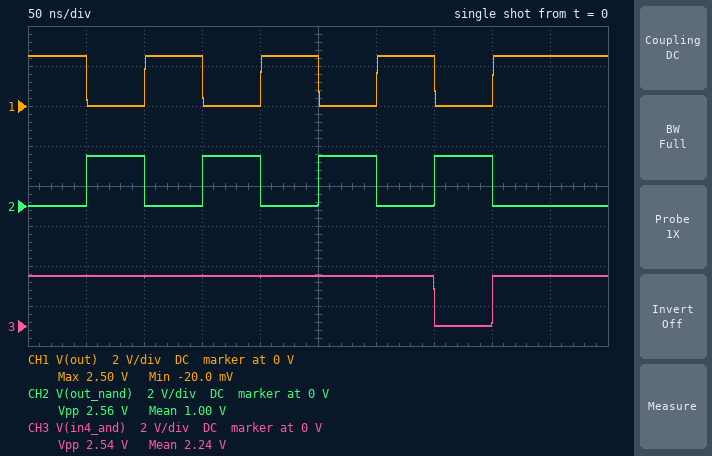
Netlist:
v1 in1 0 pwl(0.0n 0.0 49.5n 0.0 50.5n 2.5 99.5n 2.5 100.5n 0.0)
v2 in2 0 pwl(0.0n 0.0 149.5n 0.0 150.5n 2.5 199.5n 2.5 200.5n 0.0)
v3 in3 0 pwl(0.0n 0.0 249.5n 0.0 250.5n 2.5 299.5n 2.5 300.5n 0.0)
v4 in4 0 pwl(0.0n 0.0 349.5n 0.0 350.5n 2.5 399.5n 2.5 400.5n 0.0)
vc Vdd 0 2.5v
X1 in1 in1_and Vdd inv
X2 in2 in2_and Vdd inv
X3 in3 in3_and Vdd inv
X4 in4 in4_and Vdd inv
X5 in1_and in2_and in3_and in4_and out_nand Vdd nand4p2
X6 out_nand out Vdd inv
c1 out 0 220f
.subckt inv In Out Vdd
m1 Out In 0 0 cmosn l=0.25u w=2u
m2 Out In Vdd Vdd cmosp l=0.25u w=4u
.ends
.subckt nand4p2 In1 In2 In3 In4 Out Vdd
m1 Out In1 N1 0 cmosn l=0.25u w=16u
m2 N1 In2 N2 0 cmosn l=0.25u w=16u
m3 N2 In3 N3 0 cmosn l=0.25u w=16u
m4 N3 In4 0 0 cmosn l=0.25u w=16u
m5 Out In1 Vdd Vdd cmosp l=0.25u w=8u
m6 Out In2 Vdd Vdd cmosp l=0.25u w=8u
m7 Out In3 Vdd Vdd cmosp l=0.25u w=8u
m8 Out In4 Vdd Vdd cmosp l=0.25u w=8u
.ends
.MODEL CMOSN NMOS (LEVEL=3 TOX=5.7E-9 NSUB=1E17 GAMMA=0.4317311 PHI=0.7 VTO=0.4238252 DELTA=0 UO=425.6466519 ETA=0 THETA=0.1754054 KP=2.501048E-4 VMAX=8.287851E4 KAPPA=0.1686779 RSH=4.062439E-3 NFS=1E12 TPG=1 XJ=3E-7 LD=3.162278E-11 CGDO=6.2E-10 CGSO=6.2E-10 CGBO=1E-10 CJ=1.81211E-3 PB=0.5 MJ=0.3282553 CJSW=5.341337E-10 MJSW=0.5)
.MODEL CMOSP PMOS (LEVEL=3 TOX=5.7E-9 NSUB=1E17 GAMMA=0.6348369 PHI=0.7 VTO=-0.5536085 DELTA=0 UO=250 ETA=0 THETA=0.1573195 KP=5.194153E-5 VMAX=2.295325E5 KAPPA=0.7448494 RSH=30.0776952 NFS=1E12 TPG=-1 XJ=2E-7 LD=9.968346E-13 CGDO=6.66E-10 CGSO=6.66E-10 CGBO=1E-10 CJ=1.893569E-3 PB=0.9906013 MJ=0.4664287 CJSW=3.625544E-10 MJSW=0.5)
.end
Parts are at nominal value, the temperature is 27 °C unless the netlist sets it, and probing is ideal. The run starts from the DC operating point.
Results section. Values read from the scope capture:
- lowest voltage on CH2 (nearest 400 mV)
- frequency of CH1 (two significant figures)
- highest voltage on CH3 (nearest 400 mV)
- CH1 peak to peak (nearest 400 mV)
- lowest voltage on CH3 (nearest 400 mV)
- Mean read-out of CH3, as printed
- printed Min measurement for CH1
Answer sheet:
0 V
10 MHz
2.4 V
2.4 V
0 V
2.24 V
-20.0 mV
